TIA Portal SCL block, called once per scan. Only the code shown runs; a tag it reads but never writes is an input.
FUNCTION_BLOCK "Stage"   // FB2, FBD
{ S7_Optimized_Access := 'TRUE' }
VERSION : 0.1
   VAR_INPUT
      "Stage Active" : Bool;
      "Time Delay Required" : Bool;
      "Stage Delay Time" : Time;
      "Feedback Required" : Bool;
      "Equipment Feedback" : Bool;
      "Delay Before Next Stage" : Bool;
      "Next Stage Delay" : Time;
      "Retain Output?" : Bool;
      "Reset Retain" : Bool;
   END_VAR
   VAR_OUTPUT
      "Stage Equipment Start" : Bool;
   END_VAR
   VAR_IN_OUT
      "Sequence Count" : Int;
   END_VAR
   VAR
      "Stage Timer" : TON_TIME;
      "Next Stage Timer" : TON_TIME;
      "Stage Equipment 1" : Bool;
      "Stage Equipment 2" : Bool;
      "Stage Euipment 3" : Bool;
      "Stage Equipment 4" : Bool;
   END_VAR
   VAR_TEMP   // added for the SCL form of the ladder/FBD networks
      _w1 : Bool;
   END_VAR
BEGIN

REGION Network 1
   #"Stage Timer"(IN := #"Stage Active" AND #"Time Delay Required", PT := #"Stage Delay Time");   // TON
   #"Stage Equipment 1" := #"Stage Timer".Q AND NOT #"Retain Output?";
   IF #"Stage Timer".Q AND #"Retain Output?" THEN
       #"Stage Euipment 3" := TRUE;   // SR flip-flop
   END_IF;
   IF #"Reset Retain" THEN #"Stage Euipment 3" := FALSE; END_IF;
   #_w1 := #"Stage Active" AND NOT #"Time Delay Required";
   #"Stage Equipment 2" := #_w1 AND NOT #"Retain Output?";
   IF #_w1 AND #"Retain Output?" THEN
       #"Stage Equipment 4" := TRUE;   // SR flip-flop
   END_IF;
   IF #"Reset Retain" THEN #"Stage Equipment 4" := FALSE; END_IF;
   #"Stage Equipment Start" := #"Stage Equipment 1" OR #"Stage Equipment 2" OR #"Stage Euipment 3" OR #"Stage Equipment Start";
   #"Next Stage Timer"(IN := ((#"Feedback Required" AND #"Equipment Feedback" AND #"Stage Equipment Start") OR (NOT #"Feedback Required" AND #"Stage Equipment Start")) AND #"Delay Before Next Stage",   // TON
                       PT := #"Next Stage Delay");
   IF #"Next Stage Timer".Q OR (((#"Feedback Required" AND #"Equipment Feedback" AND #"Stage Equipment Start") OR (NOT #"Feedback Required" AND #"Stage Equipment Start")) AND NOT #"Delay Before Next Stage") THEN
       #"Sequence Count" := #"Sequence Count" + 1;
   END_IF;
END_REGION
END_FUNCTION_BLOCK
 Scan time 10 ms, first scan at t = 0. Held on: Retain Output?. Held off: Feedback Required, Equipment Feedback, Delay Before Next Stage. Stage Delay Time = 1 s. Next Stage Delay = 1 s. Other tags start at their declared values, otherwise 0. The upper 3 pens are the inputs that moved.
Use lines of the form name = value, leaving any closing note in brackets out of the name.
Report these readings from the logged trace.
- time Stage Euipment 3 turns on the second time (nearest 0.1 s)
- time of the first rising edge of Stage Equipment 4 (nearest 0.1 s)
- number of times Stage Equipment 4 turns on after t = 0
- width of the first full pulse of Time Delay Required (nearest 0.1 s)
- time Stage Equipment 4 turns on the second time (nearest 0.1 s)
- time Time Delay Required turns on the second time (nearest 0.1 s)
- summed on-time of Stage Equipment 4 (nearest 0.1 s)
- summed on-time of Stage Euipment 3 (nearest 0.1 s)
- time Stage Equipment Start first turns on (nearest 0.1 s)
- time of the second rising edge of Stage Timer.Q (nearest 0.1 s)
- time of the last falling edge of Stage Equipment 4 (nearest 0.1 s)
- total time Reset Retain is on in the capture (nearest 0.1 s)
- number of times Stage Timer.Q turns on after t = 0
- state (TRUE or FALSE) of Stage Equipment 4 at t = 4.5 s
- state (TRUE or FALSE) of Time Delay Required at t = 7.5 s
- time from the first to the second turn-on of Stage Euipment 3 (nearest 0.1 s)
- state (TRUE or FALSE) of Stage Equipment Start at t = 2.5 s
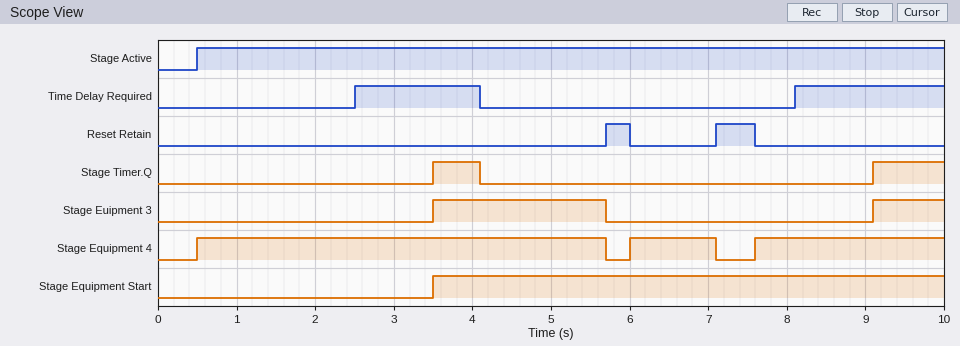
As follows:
time Stage Euipment 3 turns on the second time = 9.1 s
time of the first rising edge of Stage Equipment 4 = 0.5 s
number of times Stage Equipment 4 turns on after t = 0 = 3
width of the first full pulse of Time Delay Required = 1.6 s
time Stage Equipment 4 turns on the second time = 6.0 s
time Time Delay Required turns on the second time = 8.1 s
summed on-time of Stage Equipment 4 = 8.7 s
summed on-time of Stage Euipment 3 = 3.1 s
time Stage Equipment Start first turns on = 3.5 s
time of the second rising edge of Stage Timer.Q = 9.1 s
time of the last falling edge of Stage Equipment 4 = 7.1 s
total time Reset Retain is on in the capture = 0.8 s
number of times Stage Timer.Q turns on after t = 0 = 2
state (TRUE or FALSE) of Stage Equipment 4 at t = 4.5 s = TRUE
state (TRUE or FALSE) of Time Delay Required at t = 7.5 s = FALSE
time from the first to the second turn-on of Stage Euipment 3 = 5.6 s
state (TRUE or FALSE) of Stage Equipment Start at t = 2.5 s = FALSE
